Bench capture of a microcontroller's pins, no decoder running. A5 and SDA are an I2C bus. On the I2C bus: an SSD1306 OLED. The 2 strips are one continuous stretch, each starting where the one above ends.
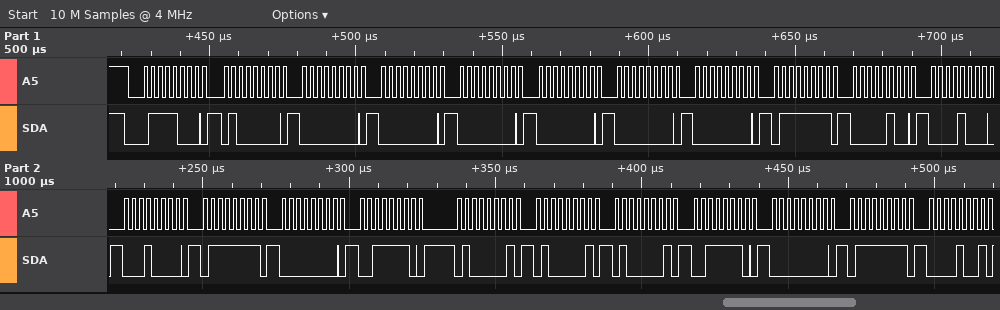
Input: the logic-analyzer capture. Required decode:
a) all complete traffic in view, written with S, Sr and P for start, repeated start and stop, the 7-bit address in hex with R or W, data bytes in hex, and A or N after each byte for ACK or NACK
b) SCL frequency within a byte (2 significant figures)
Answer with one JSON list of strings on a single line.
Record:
["S 3CW A 40 A 00 A 00 A 00 A 00 A 00 A 00 A 7F A 04 A 08 A 10 A 7F A 00 A 3E A 41 A 41 A 41 A 3E A 00 A 7F A 09 A", "400 kHz"]
